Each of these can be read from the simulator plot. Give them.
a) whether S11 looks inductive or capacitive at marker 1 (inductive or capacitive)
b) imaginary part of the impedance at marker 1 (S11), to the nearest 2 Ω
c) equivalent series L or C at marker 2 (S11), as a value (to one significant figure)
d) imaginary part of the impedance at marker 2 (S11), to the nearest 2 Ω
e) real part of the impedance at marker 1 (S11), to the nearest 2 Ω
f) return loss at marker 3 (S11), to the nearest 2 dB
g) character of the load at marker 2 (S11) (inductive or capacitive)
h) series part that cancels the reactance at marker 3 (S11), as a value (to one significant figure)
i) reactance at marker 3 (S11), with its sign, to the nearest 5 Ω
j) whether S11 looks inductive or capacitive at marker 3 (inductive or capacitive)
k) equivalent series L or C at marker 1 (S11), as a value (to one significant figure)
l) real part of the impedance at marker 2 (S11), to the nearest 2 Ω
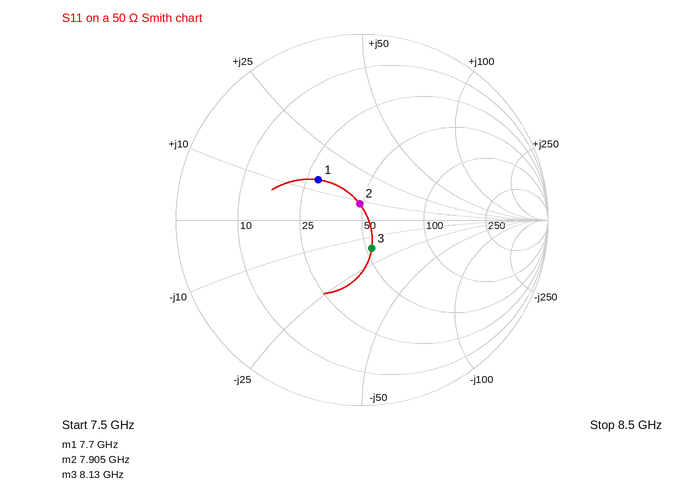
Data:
inductive
+14 Ω
200 pH
+8 Ω
28 Ω
16 dB
inductive
300 pH
-15 Ω
capacitive
300 pH
48 Ω
